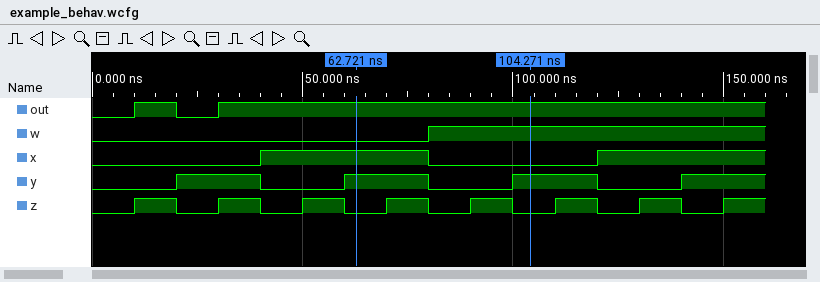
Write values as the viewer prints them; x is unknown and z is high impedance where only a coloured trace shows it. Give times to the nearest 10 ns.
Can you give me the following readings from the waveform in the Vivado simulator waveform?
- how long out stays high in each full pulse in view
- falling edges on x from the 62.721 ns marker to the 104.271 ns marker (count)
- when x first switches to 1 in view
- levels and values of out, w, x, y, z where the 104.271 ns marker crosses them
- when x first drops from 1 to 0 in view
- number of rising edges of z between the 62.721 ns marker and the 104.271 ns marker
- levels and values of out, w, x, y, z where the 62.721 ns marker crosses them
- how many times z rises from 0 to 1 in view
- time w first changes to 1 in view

10 ns
1
40 ns
out=1, w=1, x=0, y=1, z=0
80 ns
2
out=1, w=0, x=1, y=1, z=0
8
80 ns
